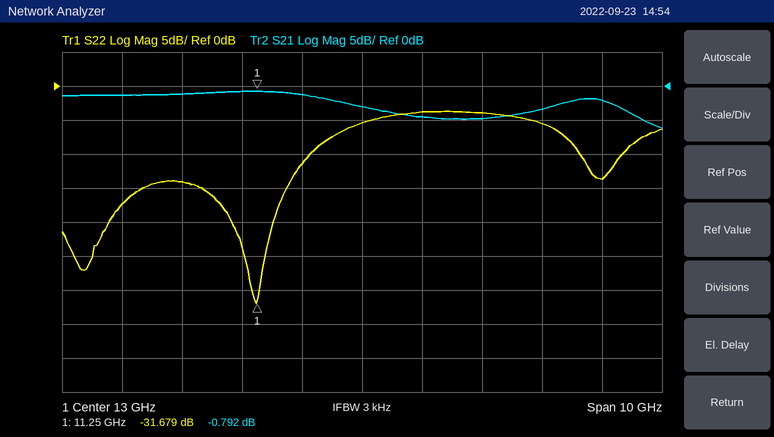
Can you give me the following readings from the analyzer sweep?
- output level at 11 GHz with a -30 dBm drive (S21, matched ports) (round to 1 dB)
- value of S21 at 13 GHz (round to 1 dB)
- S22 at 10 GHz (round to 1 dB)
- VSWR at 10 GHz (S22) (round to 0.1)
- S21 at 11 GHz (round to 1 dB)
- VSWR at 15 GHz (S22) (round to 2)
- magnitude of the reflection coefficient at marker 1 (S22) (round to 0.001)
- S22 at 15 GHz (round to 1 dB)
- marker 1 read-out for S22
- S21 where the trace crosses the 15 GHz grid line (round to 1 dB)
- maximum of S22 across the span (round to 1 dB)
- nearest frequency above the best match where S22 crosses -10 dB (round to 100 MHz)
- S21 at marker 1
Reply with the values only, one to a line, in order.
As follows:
-31 dBm
-3 dB
-14 dB
1.5
-1 dB
4
0.026
-4 dB
-31.679 dB
-5 dB
-4 dB
12.1 GHz
-0.792 dB
